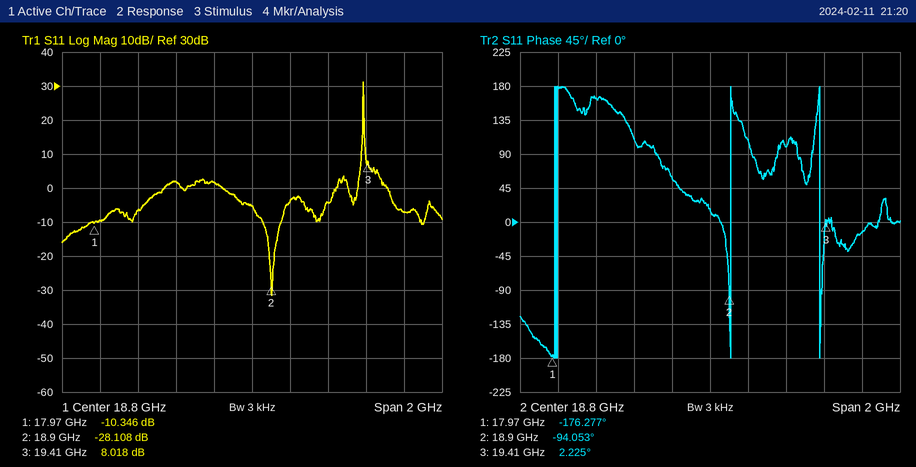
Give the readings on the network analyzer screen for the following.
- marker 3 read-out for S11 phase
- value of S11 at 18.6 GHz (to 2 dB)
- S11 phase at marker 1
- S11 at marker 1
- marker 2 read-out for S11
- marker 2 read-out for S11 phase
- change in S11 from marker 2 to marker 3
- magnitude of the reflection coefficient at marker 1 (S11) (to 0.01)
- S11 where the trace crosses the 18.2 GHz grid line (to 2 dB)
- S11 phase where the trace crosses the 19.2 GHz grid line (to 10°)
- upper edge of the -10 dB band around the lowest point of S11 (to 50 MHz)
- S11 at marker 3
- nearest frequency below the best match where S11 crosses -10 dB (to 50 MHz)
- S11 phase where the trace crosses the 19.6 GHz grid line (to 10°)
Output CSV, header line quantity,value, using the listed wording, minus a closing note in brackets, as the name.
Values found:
quantity,value
marker 3 read-out for S11 phase,2.225°
value of S11 at 18.6 GHz,2 dB
S11 phase at marker 1,-176.277°
S11 at marker 1,-10.346 dB
marker 2 read-out for S11,-28.108 dB
marker 2 read-out for S11 phase,-94.053°
change in S11 from marker 2 to marker 3,36.126 dB
magnitude of the reflection coefficient at marker 1 (S11),0.30
S11 where the trace crosses the 18.2 GHz grid line,-6 dB
S11 phase where the trace crosses the 19.2 GHz grid line,100°
upper edge of the -10 dB band around the lowest point of S11,18.95 GHz
S11 at marker 3,8.018 dB
nearest frequency below the best match where S11 crosses -10 dB,18.85 GHz
S11 phase where the trace crosses the 19.6 GHz grid line,-10°
